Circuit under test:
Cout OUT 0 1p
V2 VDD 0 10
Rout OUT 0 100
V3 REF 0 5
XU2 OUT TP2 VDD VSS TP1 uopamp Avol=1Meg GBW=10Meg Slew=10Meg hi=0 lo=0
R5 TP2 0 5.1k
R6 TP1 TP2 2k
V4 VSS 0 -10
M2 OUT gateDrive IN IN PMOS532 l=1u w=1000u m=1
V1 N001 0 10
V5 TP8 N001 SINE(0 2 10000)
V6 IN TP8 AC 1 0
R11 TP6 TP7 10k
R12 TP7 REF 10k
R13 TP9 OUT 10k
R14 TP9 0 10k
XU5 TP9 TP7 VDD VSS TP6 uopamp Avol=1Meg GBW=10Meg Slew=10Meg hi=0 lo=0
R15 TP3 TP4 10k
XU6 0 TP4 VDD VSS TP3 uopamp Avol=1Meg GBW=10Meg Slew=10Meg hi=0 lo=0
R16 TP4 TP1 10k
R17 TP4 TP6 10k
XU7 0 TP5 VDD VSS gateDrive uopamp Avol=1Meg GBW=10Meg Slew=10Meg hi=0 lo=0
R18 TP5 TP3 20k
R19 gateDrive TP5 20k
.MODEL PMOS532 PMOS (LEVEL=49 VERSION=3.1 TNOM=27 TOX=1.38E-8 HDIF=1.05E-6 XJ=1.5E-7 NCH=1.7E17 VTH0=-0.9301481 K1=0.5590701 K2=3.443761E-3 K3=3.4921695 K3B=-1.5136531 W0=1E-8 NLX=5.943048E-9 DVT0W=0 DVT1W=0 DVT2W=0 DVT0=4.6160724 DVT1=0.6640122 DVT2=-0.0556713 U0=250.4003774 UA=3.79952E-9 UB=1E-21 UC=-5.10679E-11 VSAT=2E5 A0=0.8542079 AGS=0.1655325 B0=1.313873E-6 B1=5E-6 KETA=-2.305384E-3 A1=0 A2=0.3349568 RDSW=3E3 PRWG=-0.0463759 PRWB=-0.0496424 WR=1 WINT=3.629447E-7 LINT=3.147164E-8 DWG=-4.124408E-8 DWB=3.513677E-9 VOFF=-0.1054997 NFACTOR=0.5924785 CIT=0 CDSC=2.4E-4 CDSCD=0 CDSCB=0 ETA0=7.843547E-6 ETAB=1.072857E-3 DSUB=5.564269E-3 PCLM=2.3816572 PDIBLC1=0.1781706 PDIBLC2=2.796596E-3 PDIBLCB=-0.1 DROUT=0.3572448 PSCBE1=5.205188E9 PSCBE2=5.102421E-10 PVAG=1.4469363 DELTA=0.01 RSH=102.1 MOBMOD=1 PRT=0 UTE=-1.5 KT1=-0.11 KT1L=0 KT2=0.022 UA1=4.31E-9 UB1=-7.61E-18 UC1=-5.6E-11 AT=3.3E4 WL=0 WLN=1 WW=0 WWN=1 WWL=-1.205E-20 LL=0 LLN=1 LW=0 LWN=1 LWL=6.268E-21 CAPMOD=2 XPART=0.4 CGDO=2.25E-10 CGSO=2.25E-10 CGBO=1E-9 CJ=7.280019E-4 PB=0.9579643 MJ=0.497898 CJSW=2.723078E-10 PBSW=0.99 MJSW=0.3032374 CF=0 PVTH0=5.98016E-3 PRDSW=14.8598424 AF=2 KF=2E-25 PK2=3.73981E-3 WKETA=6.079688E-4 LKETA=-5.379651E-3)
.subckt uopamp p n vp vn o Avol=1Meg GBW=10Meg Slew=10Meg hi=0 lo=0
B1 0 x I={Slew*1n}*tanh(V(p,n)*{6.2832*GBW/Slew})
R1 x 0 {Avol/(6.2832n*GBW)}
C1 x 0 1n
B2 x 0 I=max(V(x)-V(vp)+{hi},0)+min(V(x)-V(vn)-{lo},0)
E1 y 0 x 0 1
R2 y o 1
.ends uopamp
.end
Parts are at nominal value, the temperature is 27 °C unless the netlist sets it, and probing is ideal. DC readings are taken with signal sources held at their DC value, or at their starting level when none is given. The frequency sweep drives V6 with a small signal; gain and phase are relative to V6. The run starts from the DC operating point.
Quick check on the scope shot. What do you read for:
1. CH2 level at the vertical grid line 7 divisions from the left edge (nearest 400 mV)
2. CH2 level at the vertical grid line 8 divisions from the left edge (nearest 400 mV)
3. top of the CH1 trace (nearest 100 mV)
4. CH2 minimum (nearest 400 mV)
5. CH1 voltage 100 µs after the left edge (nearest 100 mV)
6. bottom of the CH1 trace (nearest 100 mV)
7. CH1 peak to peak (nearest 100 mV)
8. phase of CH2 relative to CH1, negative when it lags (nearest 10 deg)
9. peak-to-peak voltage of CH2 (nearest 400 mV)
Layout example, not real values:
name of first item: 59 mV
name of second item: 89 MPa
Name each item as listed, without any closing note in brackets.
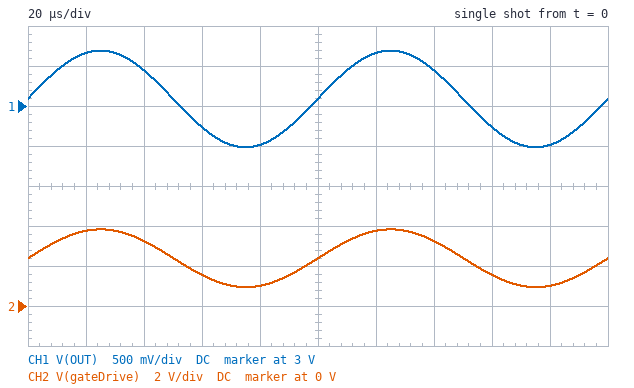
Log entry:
CH2 level at the vertical grid line 7 divisions from the left edge: 3.2 V
CH2 level at the vertical grid line 8 divisions from the left edge: 1.6 V
top of the CH1 trace: 3.7 V
CH2 minimum: 800 mV
CH1 voltage 100 µs after the left edge: 3.1 V
bottom of the CH1 trace: 2.5 V
CH1 peak to peak: 1.2 V
phase of CH2 relative to CH1, negative when it lags: 0 deg
peak-to-peak voltage of CH2: 2.8 V
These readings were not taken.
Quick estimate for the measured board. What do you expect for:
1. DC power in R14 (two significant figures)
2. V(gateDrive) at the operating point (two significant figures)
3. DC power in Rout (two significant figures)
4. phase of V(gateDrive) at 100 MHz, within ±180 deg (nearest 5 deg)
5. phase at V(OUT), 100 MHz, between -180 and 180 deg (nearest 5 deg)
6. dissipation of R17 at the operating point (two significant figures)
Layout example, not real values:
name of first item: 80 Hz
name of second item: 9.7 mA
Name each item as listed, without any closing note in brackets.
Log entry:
DC power in R14: 240 µW
V(gateDrive) at the operating point: 2.4 V
DC power in Rout: 96 mW
phase of V(gateDrive) at 100 MHz, within ±180 deg: 90 deg
phase at V(OUT), 100 MHz, between -180 and 180 deg: -5 deg
dissipation of R17 at the operating point: 360 µW
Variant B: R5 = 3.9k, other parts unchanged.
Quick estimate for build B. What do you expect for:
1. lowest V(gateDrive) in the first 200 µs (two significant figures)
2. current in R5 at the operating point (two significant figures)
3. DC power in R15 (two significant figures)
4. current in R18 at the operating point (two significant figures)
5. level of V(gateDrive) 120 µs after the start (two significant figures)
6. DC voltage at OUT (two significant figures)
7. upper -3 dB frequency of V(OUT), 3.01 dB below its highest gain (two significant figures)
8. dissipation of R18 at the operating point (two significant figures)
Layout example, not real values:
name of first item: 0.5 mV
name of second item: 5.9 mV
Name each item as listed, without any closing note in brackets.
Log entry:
lowest V(gateDrive) in the first 200 µs: 1.2 V
current in R5 at the operating point: 790 µA
DC power in R15: 740 µW
current in R18 at the operating point: 140 µA
level of V(gateDrive) 120 µs after the start: 4.1 V
DC voltage at OUT: 3.1 V
upper -3 dB frequency of V(OUT), 3.01 dB below its highest gain: 650 MHz
dissipation of R18 at the operating point: 370 µW
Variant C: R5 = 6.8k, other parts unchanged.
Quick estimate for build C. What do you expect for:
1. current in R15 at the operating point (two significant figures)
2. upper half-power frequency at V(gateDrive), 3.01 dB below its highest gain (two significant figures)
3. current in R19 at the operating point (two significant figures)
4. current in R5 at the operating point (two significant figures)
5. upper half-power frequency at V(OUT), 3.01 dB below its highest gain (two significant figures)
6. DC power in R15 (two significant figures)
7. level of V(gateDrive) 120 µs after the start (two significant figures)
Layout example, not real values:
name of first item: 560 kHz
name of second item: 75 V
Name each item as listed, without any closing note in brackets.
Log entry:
current in R15 at the operating point: 210 µA
upper half-power frequency at V(gateDrive), 3.01 dB below its highest gain: 2.5 MHz
current in R19 at the operating point: 110 µA
current in R5 at the operating point: 460 µA
upper half-power frequency at V(OUT), 3.01 dB below its highest gain: 720 MHz
DC power in R15: 450 µW
level of V(gateDrive) 120 µs after the start: 3.4 V
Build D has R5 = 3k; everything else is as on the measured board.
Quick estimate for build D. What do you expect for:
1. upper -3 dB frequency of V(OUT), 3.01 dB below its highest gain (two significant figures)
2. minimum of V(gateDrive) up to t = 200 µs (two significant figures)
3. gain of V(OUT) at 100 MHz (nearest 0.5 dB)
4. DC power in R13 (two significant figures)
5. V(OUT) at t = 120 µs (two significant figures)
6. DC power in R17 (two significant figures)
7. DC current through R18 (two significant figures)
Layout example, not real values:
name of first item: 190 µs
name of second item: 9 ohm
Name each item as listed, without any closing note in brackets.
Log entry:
upper -3 dB frequency of V(OUT), 3.01 dB below its highest gain: 580 MHz
minimum of V(gateDrive) up to t = 200 µs: 1.6 V
gain of V(OUT) at 100 MHz: -9.0 dB
DC power in R13: 230 µW
V(OUT) at t = 120 µs: 3.6 V
DC power in R17: 380 µW
DC current through R18: 160 µA
